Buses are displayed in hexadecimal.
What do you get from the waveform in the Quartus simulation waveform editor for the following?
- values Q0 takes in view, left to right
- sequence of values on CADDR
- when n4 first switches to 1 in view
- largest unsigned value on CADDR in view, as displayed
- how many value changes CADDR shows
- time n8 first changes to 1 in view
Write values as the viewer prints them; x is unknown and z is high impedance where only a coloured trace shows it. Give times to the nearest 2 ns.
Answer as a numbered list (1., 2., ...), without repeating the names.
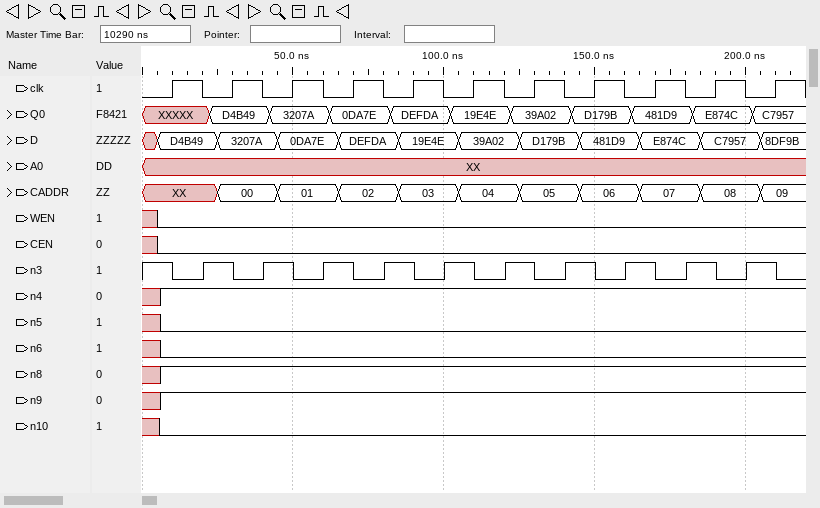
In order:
1. XXXXX, D4B49, 3207A, 0DA7E, DEFDA, 19E4E, 39A02, D179B, 481D9, E874C, C7957
2. XX, 00, 01, 02, 03, 04, 05, 06, 07, 08, 09
3. 6 ns
4. 09
5. 10
6. 6 ns
